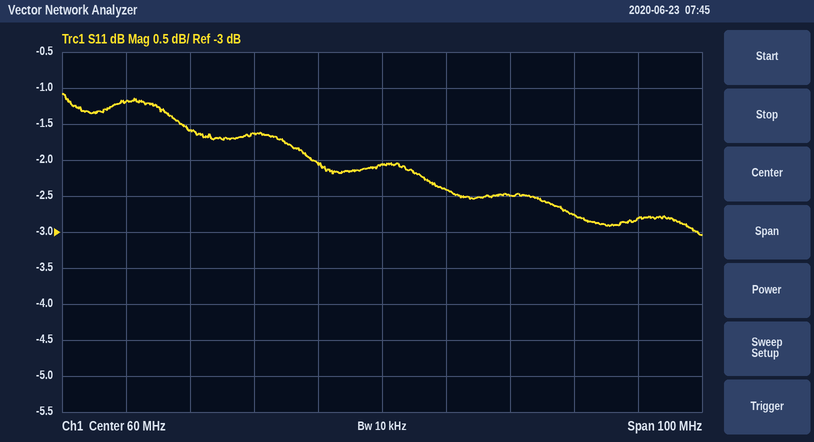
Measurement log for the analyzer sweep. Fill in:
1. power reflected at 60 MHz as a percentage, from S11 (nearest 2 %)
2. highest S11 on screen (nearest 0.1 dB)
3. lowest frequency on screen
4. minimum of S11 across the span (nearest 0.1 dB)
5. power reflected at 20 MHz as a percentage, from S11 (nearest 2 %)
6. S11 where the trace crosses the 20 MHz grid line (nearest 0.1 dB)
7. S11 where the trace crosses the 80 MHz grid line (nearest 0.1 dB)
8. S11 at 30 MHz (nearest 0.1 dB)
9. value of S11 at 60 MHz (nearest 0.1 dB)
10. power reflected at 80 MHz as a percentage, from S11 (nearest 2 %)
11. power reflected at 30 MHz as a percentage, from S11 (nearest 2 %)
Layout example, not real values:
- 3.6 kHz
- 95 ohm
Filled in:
- 62 %
- -1.1 dB
- 10 MHz
- -3.0 dB
- 76 %
- -1.2 dB
- -2.5 dB
- -1.6 dB
- -2.1 dB
- 56 %
- 70 %
